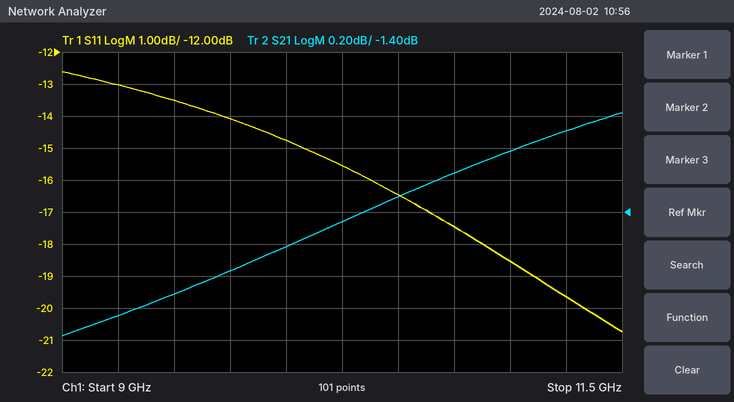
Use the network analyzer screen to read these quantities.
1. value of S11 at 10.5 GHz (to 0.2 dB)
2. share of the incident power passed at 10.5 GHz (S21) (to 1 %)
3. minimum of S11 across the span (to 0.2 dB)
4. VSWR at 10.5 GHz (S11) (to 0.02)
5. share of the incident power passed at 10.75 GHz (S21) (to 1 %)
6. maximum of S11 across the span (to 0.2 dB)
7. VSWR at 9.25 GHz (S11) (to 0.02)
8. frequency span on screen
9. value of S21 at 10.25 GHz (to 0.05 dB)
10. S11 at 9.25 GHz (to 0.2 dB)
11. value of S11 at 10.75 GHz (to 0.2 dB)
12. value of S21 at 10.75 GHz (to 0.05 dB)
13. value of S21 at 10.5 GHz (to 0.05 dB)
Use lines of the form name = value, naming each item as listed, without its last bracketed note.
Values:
value of S11 at 10.5 GHz = -16.4 dB
share of the incident power passed at 10.5 GHz (S21) = 74 %
minimum of S11 across the span = -20.8 dB
VSWR at 10.5 GHz (S11) = 1.36
share of the incident power passed at 10.75 GHz (S21) = 77 %
maximum of S11 across the span = -12.6 dB
VSWR at 9.25 GHz (S11) = 1.58
frequency span on screen = 2.5 GHz
value of S21 at 10.25 GHz = -1.45 dB
S11 at 9.25 GHz = -13.0 dB
value of S11 at 10.75 GHz = -17.4 dB
value of S21 at 10.75 GHz = -1.15 dB
value of S21 at 10.5 GHz = -1.30 dB
